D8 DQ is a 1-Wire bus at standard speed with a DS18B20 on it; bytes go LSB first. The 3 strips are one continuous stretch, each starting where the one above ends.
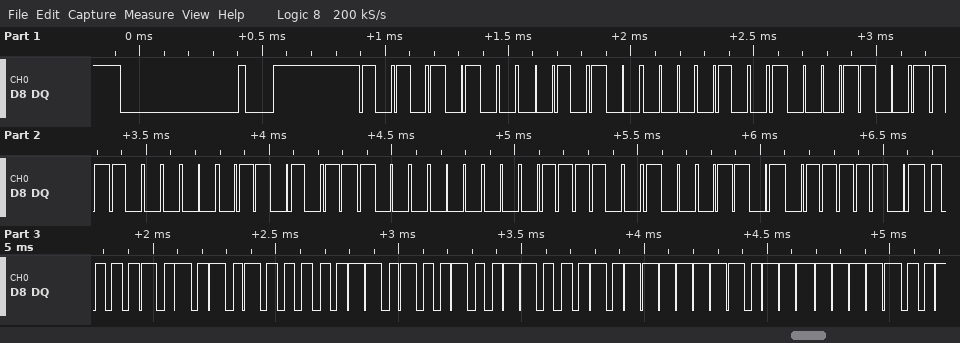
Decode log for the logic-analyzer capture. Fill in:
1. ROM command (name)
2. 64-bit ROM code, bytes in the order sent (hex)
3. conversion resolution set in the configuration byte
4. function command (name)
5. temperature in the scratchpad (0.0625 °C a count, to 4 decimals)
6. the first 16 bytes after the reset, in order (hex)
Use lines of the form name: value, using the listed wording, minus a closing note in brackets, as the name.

ROM command: Match ROM
64-bit ROM code, bytes in the order sent: 28 90 98 07 D6 01 3C B1
conversion resolution set in the configuration byte: 12 bits
function command: Read Scratchpad
temperature in the scratchpad: 85.0000 °C
the first 16 bytes after the reset, in order: 55 28 90 98 07 D6 01 3C B1 BE 50 05 4B 46 7F FF
